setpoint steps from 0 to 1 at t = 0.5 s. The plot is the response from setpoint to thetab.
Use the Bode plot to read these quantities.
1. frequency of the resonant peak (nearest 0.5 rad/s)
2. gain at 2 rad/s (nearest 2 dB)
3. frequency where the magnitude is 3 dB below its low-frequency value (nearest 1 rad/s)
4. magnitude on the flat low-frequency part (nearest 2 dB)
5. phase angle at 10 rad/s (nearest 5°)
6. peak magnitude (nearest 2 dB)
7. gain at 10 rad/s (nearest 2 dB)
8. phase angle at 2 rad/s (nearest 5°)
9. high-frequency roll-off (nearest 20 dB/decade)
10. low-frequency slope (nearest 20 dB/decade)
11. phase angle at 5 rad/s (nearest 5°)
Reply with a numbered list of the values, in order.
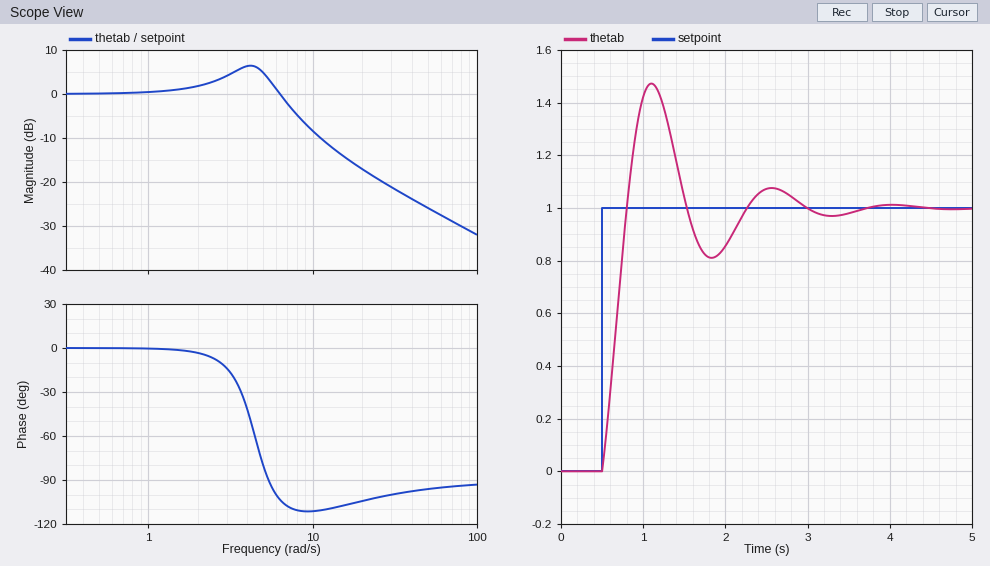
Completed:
1. 4.0 rad/s
2. 2 dB
3. 7 rad/s
4. 0 dB
5. -110°
6. 6 dB
7. -8 dB
8. -5°
9. -20 dB/decade
10. 0 dB/decade
11. -80°
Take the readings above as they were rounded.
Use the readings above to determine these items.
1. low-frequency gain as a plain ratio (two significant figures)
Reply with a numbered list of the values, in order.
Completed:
1. 1.0
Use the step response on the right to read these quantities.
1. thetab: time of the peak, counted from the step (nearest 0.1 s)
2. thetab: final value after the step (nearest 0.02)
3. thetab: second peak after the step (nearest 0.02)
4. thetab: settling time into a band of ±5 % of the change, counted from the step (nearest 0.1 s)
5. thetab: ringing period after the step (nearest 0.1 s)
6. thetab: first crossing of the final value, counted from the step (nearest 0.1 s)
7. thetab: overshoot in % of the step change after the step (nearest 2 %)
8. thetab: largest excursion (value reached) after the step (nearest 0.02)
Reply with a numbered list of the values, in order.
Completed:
1. 0.6 s
2. 1.00
3. 1.08
4. 2.3 s
5. 1.5 s
6. 0.3 s
7. 48 %
8. 1.48
